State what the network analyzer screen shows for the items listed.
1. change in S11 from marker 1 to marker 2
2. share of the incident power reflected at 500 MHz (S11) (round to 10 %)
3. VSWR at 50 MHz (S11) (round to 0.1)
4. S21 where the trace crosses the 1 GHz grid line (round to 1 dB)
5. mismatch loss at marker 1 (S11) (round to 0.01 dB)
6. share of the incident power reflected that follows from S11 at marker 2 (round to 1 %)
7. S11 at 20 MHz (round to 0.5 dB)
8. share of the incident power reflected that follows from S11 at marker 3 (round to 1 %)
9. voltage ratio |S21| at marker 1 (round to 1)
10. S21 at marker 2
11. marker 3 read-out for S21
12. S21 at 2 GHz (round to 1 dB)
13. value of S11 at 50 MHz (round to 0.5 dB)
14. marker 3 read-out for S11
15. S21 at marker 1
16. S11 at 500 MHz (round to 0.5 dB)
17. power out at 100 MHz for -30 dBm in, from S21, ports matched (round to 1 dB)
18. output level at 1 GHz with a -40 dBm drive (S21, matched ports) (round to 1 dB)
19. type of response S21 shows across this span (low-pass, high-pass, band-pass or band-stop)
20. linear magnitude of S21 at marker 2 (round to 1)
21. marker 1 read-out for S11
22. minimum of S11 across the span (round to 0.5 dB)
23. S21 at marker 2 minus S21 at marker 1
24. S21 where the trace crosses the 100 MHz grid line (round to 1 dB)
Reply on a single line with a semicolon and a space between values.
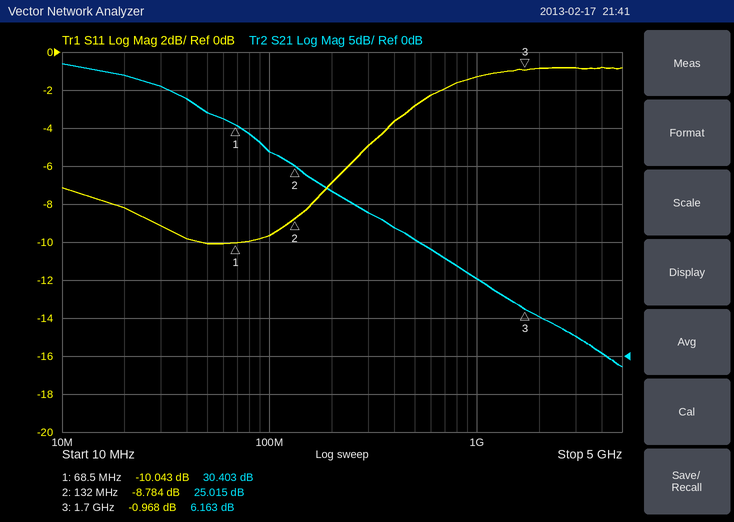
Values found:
1.259 dB; 50 %; 1.9; 10 dB; 0.45 dB; 13 %; -8.0 dB; 80 %; 33; 25.015 dB; 6.163 dB; 5 dB; -10.0 dB; -0.968 dB; 30.403 dB; -3.0 dB; -3 dBm; -30 dBm; low-pass; 18; -10.043 dB; -10.0 dB; -5.388 dB; 27 dB
